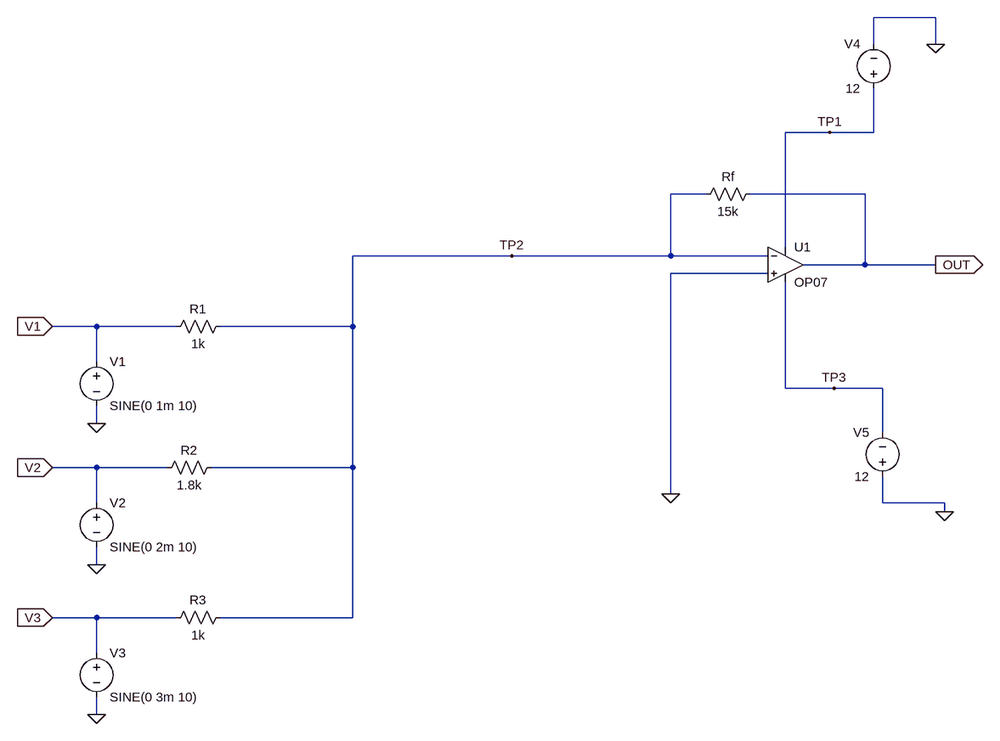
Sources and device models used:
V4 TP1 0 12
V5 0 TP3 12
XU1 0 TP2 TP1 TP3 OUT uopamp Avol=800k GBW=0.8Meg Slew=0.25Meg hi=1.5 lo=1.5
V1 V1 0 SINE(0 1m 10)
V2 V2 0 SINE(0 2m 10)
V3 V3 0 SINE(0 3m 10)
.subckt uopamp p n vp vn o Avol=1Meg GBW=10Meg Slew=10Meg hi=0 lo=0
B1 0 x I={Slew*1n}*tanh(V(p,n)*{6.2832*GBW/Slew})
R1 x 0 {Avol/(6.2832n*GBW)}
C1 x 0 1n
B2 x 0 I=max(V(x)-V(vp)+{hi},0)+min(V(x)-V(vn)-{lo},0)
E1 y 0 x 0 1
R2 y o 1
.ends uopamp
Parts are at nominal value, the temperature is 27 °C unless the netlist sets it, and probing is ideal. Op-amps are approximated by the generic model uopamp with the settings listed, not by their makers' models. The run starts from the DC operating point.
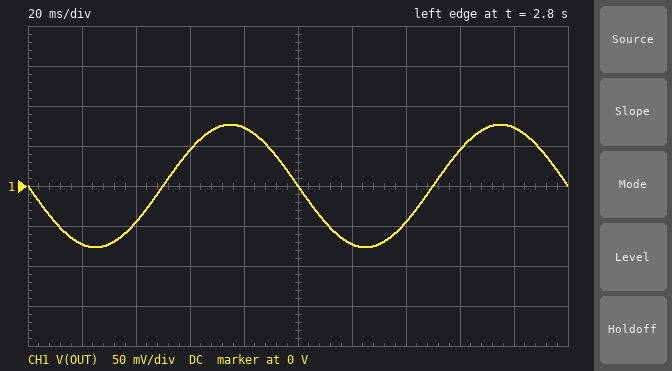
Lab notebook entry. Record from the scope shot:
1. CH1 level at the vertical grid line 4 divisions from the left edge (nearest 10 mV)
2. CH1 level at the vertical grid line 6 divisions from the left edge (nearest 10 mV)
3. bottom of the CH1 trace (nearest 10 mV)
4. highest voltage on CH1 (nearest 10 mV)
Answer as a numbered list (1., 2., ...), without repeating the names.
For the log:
1. 70 mV
2. -70 mV
3. -80 mV
4. 80 mV
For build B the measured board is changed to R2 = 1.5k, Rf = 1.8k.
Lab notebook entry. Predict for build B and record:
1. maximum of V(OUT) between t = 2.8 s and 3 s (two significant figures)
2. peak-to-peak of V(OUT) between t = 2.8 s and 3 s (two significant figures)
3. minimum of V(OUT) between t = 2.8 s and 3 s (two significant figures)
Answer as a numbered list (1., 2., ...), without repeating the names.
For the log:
1. 9.6 mV
2. 19 mV
3. -9.6 mV
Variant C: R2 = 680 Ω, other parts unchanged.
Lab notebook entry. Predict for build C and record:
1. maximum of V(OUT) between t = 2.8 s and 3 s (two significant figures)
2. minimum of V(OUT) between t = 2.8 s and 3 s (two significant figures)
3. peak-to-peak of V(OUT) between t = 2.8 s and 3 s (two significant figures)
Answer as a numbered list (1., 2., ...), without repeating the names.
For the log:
1. 100 mV
2. -100 mV
3. 210 mV
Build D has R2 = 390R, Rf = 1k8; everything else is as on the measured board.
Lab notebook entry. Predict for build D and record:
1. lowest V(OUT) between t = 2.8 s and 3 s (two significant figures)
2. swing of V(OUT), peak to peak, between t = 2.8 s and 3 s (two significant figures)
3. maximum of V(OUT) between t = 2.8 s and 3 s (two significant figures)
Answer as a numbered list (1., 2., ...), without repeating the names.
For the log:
1. -16 mV
2. 33 mV
3. 16 mV
